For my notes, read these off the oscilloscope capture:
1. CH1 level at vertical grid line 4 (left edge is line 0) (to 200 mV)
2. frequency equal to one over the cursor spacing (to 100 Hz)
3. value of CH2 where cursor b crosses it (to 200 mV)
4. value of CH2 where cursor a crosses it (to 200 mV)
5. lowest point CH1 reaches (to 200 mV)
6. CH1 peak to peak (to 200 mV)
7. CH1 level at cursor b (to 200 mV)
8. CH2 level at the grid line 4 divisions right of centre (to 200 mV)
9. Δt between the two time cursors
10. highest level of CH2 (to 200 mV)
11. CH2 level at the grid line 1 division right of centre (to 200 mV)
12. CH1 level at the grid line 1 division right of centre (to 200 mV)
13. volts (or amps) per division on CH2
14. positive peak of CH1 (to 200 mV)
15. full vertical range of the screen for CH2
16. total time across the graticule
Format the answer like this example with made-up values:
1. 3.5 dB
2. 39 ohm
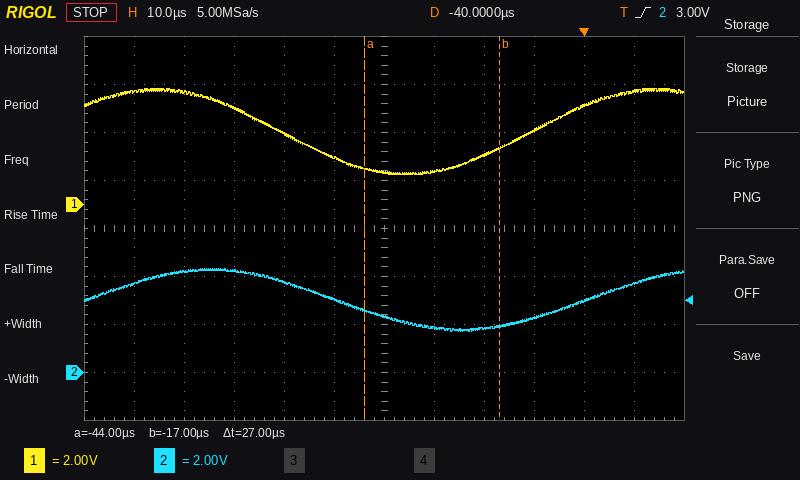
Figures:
1. 3.0 V
2. 37.0 kHz
3. 2.0 V
4. 2.6 V
5. 1.2 V
6. 3.6 V
7. 2.4 V
8. 3.0 V
9. 27 µs
10. 4.4 V
11. 1.8 V
12. 1.4 V
13. 2 V
14. 4.8 V
15. 16 V
16. 120 µs
